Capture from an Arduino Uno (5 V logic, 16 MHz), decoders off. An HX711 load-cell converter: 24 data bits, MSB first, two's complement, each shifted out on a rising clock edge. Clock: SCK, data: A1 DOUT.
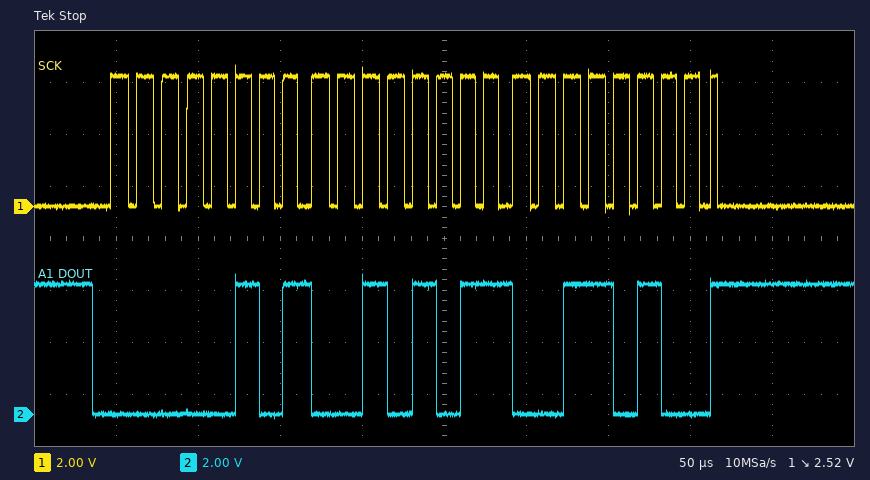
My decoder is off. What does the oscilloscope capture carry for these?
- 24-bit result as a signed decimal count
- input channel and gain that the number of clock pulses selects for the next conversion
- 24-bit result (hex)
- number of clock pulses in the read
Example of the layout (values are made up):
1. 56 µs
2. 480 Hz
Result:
1. 338740
2. channel A, gain 128
3. 0x052B34
4. 25
